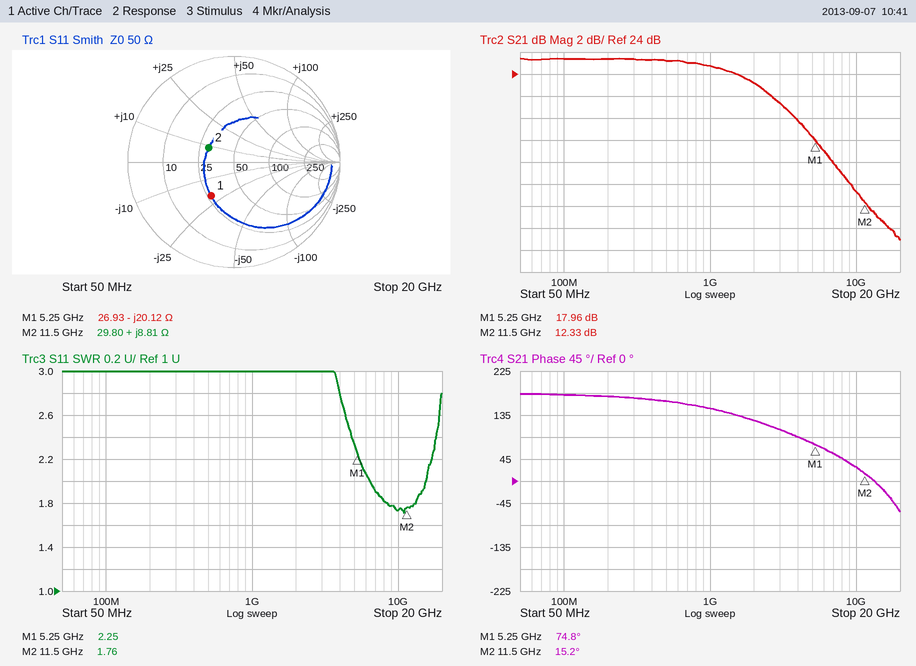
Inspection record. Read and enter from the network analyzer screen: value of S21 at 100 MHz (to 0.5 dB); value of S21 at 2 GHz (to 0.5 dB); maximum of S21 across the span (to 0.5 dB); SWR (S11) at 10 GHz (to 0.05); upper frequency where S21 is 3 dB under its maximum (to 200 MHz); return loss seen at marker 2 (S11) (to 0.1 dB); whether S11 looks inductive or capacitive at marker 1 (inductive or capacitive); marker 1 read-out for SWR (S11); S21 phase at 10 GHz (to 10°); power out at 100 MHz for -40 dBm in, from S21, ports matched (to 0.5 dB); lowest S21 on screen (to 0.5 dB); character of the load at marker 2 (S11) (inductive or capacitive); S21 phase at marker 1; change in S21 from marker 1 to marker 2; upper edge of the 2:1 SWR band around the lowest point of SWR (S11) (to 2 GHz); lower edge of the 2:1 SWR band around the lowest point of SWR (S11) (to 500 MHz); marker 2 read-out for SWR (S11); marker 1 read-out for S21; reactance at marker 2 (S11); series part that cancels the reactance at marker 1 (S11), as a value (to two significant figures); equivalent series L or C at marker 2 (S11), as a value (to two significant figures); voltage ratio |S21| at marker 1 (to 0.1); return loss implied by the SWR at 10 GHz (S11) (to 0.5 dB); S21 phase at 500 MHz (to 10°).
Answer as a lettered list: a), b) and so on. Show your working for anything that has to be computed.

a) 25.5 dB
b) 23.0 dB
c) 25.5 dB
d) 1.75
e) 2.4 GHz
f) 11.2 dB
g) capacitive
h) 2.25
i) 30°
j) -40 dBm + (25.5 dB) = -14.5 dBm
k) 9.0 dB
l) inductive
m) 74.8°
n) 12.33 − (17.96) = -5.63 dB
o) 16 GHz
p) 6.5 GHz
q) 1.76
r) 17.96 dB
s) +8.81 Ω
t) L = 20.12 Ω/(2π × 5.25 GHz) ≈ 610 pH
u) L = 8.81 Ω/(2π × 11.5 GHz) ≈ 122 pH, so 120 pH to two significant figures
v) 10^(17.96/20) ≈ 7.9
w) −20 log10((1.75 − 1)/(1.75 + 1)) ≈ 11.3 dB, so 11.5 dB to the nearest 0.5 dB
x) 160°
